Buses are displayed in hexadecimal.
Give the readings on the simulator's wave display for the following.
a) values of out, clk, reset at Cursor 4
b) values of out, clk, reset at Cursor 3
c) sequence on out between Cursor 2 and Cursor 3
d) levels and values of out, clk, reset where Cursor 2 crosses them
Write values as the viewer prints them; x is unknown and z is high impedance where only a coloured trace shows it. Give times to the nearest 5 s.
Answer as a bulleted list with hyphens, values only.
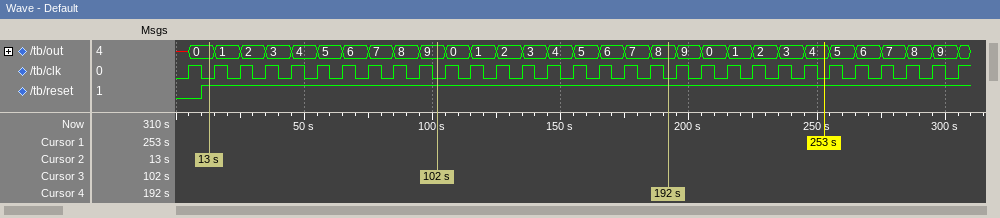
- out=8, clk=0, reset=1
- out=9, clk=0, reset=1
- 0, 1, 2, 3, 4, 5, 6, 7, 8, 9
- out=0, clk=0, reset=1
